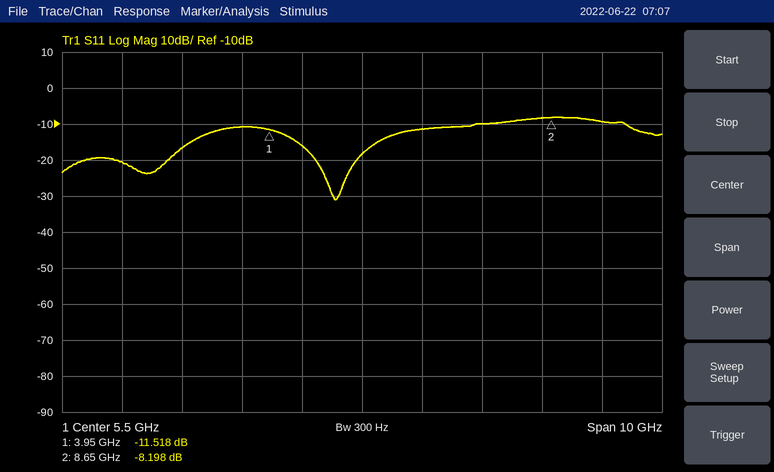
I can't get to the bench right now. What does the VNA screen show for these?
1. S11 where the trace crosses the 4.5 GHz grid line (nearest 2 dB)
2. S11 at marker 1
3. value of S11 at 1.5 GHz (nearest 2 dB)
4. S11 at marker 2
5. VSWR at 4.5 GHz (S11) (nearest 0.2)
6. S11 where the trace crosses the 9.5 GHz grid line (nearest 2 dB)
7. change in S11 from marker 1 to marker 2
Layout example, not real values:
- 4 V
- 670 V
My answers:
- -16 dB
- -11.518 dB
- -20 dB
- -8.198 dB
- 1.4
- -10 dB
- 3.320 dB
